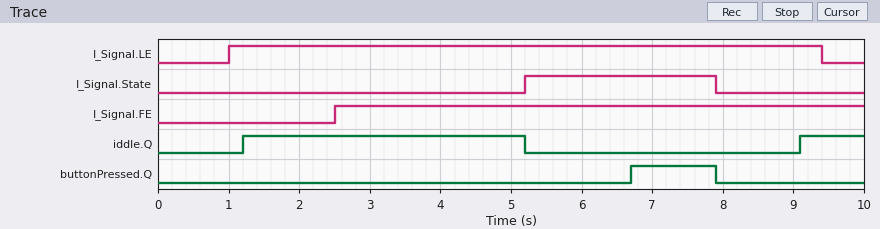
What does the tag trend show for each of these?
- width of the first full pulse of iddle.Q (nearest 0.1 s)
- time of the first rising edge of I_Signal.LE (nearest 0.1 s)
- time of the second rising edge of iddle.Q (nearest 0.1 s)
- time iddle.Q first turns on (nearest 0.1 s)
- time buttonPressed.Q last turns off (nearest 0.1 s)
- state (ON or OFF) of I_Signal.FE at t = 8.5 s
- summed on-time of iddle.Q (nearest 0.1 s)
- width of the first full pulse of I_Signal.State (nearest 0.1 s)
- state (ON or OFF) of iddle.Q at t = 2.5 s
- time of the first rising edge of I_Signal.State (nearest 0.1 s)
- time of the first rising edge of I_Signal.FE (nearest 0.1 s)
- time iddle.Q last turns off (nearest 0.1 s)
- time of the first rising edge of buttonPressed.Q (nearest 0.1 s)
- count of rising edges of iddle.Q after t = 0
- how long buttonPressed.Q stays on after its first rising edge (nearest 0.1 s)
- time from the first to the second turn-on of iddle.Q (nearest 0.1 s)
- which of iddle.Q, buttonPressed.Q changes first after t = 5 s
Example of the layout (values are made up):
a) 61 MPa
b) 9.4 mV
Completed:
a) 4.0 s
b) 1.0 s
c) 9.1 s
d) 1.2 s
e) 7.9 s
f) ON
g) 4.9 s
h) 2.7 s
i) ON
j) 5.2 s
k) 2.5 s
l) 5.2 s
m) 6.7 s
n) 2
o) 1.2 s
p) 7.9 s
q) iddle.Q
